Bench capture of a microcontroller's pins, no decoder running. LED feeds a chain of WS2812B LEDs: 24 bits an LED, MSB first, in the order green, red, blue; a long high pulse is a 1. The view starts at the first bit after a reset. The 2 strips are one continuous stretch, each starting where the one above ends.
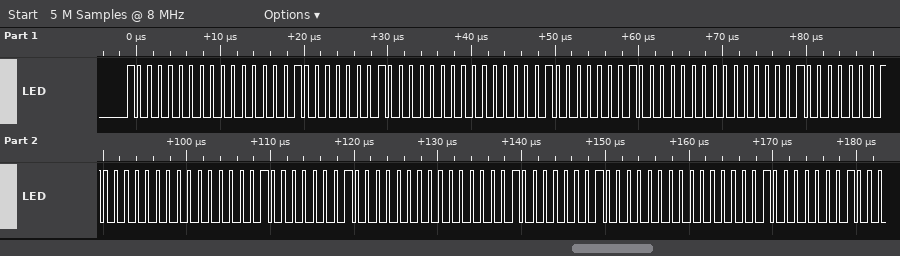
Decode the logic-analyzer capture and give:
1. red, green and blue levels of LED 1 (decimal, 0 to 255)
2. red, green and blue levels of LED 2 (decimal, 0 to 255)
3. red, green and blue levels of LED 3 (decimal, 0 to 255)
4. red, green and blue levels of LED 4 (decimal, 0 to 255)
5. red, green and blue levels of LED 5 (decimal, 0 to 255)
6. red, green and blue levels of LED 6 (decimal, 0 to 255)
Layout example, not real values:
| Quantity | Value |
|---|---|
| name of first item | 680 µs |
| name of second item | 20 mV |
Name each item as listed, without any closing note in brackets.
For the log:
| Quantity | Value |
|---|---|
| red, green and blue levels of LED 1 | 0, 128, 128 |
| red, green and blue levels of LED 2 | 0, 128, 128 |
| red, green and blue levels of LED 3 | 0, 128, 128 |
| red, green and blue levels of LED 4 | 0, 128, 128 |
| red, green and blue levels of LED 5 | 0, 128, 128 |
| red, green and blue levels of LED 6 | 0, 128, 128 |
